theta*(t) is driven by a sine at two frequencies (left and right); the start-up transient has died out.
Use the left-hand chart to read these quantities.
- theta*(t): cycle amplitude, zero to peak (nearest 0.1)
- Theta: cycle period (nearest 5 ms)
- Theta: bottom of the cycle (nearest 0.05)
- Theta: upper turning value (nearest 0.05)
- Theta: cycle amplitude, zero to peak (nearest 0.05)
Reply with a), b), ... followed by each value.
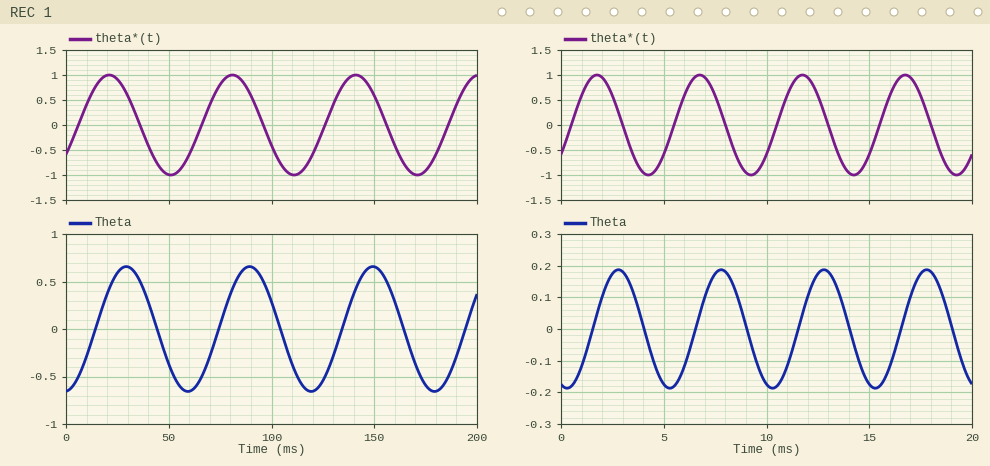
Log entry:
a) 1.0
b) 60 ms
c) -0.65
d) 0.65
e) 0.65
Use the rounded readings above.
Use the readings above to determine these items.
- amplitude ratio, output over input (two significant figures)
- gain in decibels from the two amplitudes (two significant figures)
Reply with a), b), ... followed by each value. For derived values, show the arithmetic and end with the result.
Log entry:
a) 0.65 / 1 = 0.65
b) 20 log10(0.65 / 1) = -3.7 dB
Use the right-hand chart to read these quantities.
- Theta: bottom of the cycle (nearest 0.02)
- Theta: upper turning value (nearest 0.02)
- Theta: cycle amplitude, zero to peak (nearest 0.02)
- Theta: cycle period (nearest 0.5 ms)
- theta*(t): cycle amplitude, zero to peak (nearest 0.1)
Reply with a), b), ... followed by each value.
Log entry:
a) -0.18
b) 0.18
c) 0.18
d) 5.0 ms
e) 1.0
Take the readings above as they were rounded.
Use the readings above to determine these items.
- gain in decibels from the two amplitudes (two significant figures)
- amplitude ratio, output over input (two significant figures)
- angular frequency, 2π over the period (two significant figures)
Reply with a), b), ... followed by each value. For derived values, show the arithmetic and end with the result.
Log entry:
a) 20 log10(0.18 / 1) = -15 dB
b) 0.18 / 1 = 0.18
c) 2π / 5 = 1.3 rad/ms
